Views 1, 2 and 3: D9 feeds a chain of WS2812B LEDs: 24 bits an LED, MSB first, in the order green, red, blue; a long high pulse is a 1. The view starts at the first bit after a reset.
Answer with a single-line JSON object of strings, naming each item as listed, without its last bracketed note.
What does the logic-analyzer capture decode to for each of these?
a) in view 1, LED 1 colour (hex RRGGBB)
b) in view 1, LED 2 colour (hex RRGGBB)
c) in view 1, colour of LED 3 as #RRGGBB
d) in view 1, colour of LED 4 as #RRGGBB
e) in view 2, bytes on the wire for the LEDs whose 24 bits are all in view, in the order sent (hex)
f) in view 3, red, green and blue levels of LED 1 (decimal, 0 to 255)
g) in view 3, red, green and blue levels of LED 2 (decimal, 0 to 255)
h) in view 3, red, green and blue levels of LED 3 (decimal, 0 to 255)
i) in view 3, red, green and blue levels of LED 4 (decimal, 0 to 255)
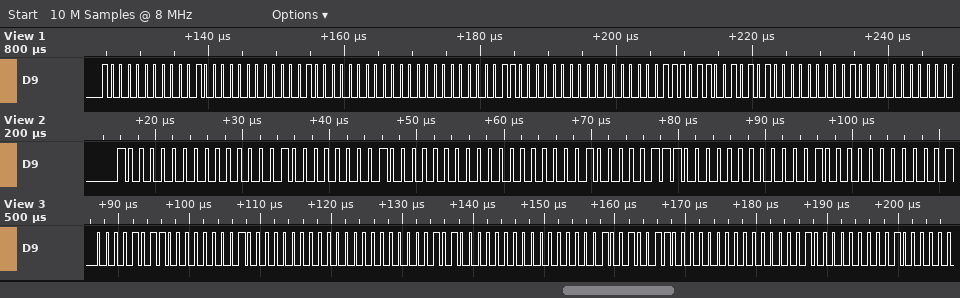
{"in view 1, LED 1 colour": "#108000", "in view 1, LED 2 colour": "#008001", "in view 1, colour of LED 3 as #RRGGBB": "#00803B", "in view 1, colour of LED 4 as #RRGGBB": "#002A80", "in view 2, bytes on the wire for the LEDs whose 24 bits are all in view, in the order sent": "80 01 00 80 00 10 70 00 80", "in view 3, red, green and blue levels of LED 1": "0, 11, 128", "in view 3, red, green and blue levels of LED 2": "2, 0, 128", "in view 3, red, green and blue levels of LED 3": "73, 0, 128", "in view 3, red, green and blue levels of LED 4": "128, 0, 32"}
